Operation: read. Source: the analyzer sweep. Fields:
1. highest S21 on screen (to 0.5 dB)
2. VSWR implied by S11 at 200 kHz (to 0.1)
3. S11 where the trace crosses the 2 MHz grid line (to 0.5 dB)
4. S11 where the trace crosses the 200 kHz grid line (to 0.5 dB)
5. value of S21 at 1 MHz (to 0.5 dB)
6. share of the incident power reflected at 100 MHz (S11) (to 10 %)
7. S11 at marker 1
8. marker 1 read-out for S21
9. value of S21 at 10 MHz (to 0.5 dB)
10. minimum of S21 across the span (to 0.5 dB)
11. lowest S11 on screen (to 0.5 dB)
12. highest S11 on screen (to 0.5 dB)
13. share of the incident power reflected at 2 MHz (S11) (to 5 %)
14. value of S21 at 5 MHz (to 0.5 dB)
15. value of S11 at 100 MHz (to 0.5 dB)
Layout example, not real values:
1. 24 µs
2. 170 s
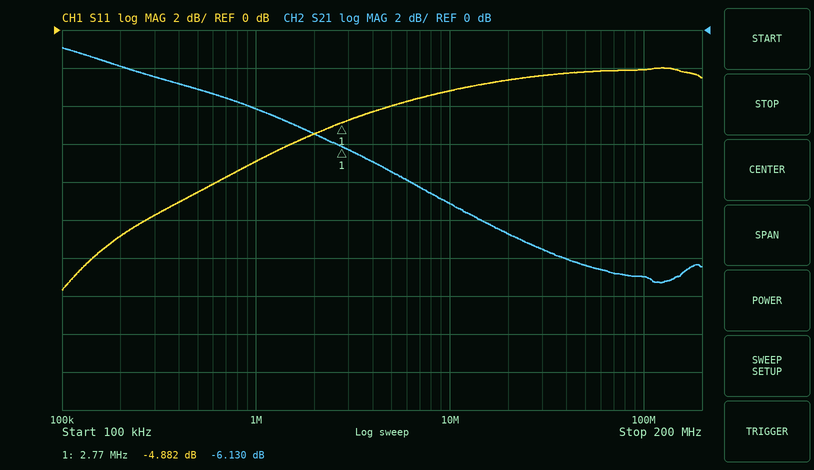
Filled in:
1. -1.0 dB
2. 1.8
3. -5.5 dB
4. -11.0 dB
5. -4.0 dB
6. 60 %
7. -4.882 dB
8. -6.130 dB
9. -9.0 dB
10. -13.5 dB
11. -13.5 dB
12. -2.0 dB
13. 30 %
14. -7.5 dB
15. -2.0 dB
